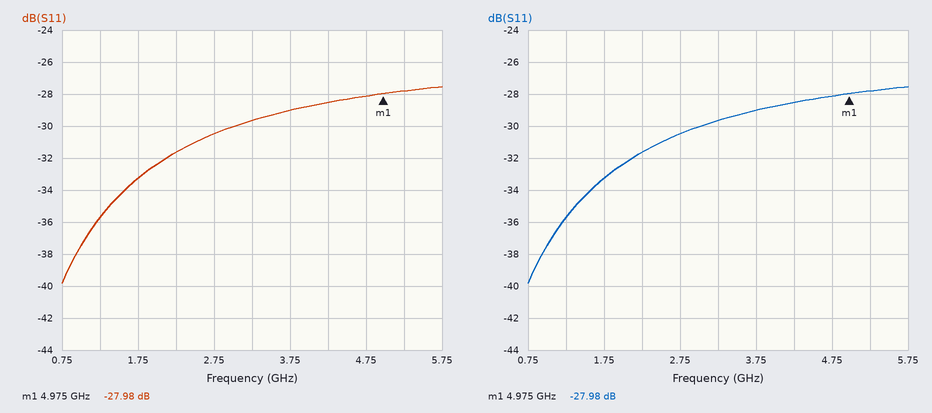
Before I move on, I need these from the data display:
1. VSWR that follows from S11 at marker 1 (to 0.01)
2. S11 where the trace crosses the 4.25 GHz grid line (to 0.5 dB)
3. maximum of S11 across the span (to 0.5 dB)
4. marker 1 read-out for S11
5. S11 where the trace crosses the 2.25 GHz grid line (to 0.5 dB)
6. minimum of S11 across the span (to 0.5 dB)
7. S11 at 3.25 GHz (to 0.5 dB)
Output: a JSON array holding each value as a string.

["1.08", "-28.5 dB", "-27.5 dB", "-27.98 dB", "-31.5 dB", "-40.0 dB", "-29.5 dB"]
